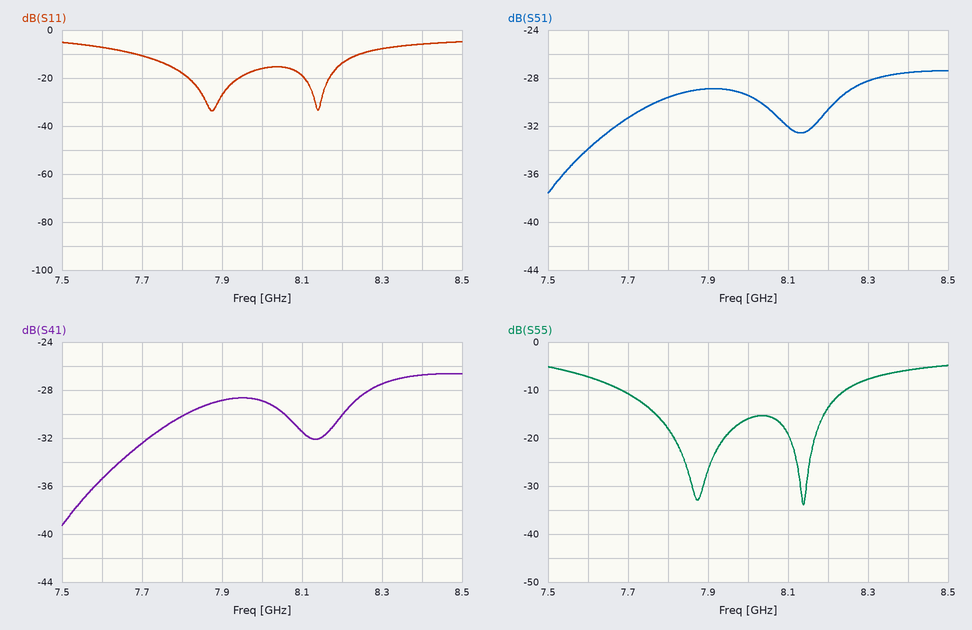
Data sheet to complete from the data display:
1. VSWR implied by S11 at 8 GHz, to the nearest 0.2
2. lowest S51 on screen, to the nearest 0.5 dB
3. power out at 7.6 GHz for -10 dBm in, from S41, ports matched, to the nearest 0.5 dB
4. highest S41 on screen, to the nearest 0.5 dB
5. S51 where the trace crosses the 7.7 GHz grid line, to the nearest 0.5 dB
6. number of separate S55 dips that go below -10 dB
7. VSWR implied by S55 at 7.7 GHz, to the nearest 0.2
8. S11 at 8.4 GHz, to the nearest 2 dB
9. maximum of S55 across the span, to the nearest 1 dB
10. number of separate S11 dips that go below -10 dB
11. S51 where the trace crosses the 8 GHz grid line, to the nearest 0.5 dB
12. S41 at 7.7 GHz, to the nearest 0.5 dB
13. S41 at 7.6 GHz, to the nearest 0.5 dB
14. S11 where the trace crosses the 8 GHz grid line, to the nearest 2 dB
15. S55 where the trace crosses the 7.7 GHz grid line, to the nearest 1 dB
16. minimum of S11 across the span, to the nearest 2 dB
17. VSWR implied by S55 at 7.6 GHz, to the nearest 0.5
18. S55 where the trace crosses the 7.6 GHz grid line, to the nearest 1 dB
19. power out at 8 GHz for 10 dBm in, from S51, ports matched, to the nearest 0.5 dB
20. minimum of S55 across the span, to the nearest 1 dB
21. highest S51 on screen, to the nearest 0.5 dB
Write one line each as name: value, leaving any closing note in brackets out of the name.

VSWR implied by S11 at 8 GHz, to the nearest 0.2: 1.4
lowest S51 on screen, to the nearest 0.5 dB: -37.5 dB
power out at 7.6 GHz for -10 dBm in, from S41, ports matched, to the nearest 0.5 dB: -45.5 dBm
highest S41 on screen, to the nearest 0.5 dB: -26.5 dB
S51 where the trace crosses the 7.7 GHz grid line, to the nearest 0.5 dB: -31.5 dB
number of separate S55 dips that go below -10 dB: 2
VSWR implied by S55 at 7.7 GHz, to the nearest 0.2: 1.8
S11 at 8.4 GHz, to the nearest 2 dB: -6 dB
maximum of S55 across the span, to the nearest 1 dB: -5 dB
number of separate S11 dips that go below -10 dB: 2
S51 where the trace crosses the 8 GHz grid line, to the nearest 0.5 dB: -29.5 dB
S41 at 7.7 GHz, to the nearest 0.5 dB: -32.5 dB
S41 at 7.6 GHz, to the nearest 0.5 dB: -35.5 dB
S11 where the trace crosses the 8 GHz grid line, to the nearest 2 dB: -16 dB
S55 where the trace crosses the 7.7 GHz grid line, to the nearest 1 dB: -11 dB
minimum of S11 across the span, to the nearest 2 dB: -34 dB
VSWR implied by S55 at 7.6 GHz, to the nearest 0.5: 2.5
S55 where the trace crosses the 7.6 GHz grid line, to the nearest 1 dB: -7 dB
power out at 8 GHz for 10 dBm in, from S51, ports matched, to the nearest 0.5 dB: -19.5 dBm
minimum of S55 across the span, to the nearest 1 dB: -34 dB
highest S51 on screen, to the nearest 0.5 dB: -27.5 dB
